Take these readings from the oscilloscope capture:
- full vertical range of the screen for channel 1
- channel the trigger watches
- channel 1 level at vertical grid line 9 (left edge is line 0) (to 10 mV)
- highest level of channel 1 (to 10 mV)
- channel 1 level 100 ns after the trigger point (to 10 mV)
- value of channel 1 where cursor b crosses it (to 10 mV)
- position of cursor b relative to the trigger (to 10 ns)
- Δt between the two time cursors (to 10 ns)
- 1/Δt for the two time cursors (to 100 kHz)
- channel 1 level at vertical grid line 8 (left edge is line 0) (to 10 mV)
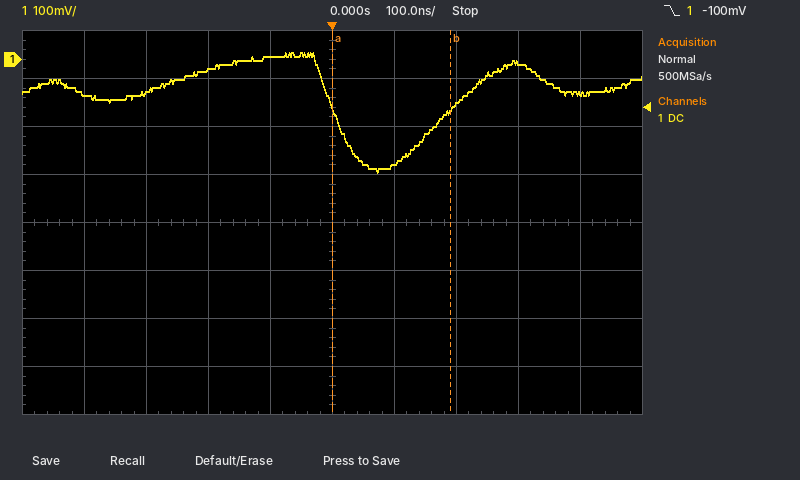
800 mV
channel 1
-70 mV
10 mV
-220 mV
-110 mV
+190 ns
190 ns
5.3 MHz
-10 mV
